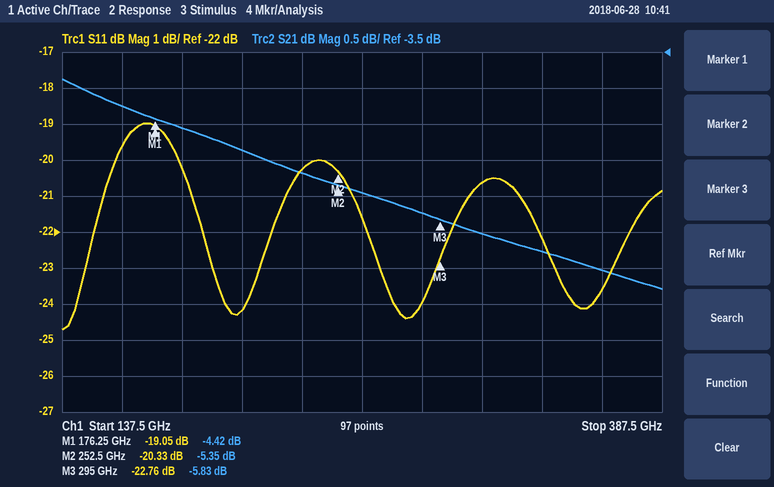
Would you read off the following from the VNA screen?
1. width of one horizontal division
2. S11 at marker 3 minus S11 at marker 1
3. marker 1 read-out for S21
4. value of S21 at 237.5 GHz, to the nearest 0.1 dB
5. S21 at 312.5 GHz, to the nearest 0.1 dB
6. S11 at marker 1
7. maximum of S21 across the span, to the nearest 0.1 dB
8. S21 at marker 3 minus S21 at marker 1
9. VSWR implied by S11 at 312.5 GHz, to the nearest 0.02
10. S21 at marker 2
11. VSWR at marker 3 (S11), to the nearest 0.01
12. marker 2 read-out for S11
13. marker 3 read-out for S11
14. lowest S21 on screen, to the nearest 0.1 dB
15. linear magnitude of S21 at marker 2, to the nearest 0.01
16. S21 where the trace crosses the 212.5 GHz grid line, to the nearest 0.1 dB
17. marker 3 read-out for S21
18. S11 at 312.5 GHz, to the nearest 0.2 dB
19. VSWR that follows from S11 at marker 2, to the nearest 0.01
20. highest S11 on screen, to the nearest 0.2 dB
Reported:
25 GHz
-3.71 dB
-4.42 dB
-5.2 dB
-6.0 dB
-19.05 dB
-3.9 dB
-1.41 dB
1.20
-5.35 dB
1.16
-20.33 dB
-22.76 dB
-6.8 dB
0.54
-4.9 dB
-5.83 dB
-20.6 dB
1.21
-19.0 dB
